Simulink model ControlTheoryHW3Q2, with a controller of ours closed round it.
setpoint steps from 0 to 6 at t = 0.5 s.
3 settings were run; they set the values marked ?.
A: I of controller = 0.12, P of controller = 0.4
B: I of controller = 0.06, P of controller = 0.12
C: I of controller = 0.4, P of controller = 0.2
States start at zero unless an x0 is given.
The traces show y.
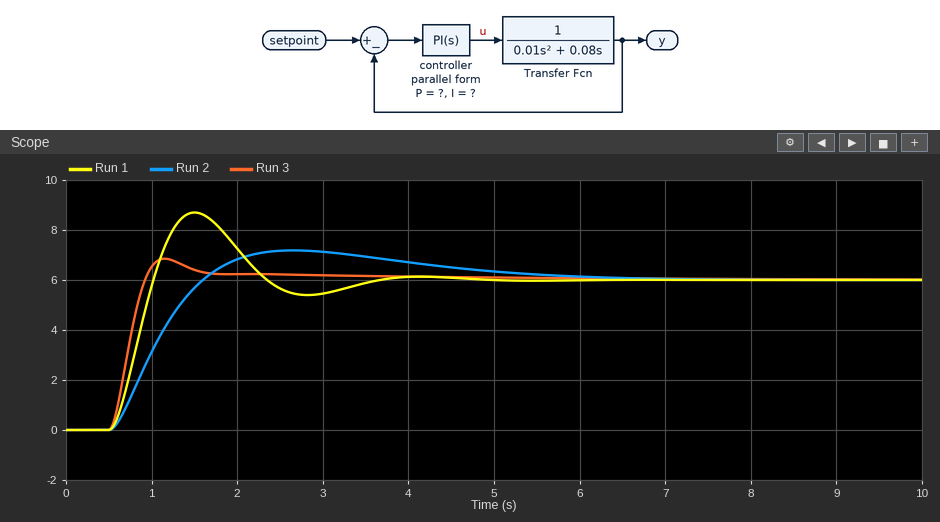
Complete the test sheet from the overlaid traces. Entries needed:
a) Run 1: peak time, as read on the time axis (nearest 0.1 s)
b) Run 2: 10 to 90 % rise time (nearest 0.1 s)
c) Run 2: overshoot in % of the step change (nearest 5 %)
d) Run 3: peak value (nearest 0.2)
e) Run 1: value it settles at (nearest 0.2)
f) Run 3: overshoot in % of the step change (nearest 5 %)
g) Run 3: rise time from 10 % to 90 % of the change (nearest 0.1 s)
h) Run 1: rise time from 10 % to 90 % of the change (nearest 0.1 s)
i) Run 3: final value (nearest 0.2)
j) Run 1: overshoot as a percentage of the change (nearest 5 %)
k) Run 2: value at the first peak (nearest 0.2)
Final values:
1.5 s
0.8 s
20 %
6.8
6.0
15 %
0.3 s
0.4 s
6.0
45 %
7.2
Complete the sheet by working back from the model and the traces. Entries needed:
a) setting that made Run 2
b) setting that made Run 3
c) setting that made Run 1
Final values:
B
A
C
